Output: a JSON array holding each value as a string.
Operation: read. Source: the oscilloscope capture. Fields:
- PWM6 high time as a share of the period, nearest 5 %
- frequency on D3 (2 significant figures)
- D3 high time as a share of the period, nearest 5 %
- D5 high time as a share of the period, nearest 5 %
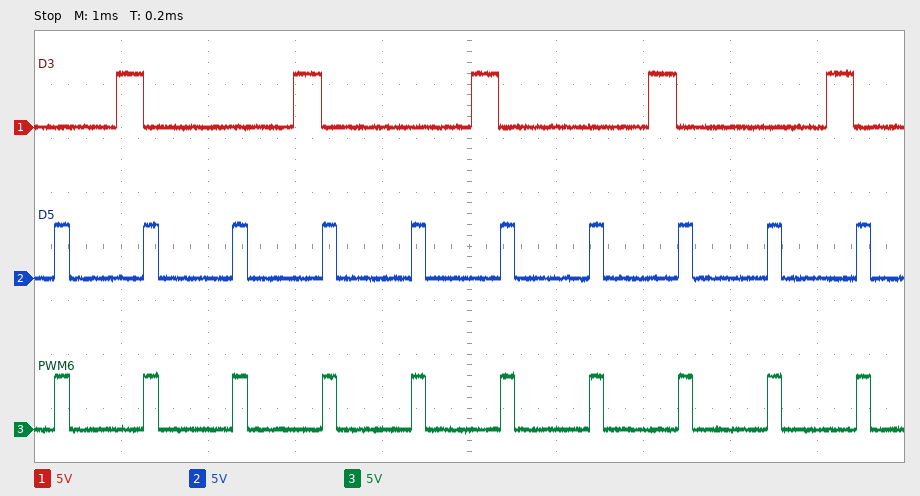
["15 %", "490 Hz", "15 %", "15 %"]
